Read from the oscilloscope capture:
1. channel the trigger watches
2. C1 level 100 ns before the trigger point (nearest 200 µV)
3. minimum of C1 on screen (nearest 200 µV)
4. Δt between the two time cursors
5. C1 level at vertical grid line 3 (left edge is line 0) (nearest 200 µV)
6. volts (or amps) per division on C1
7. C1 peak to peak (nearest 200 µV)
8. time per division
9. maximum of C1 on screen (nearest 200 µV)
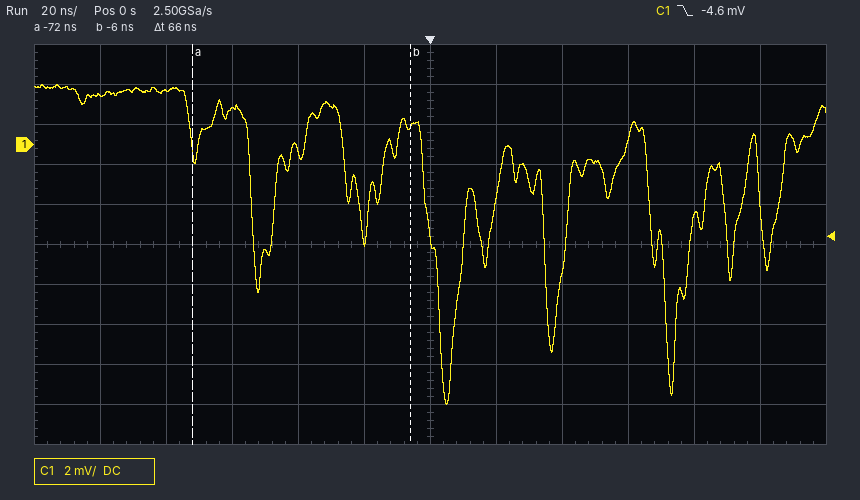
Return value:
C1
2.4 mV
-13.0 mV
66 ns
1.8 mV
2 mV
16.0 mV
20 ns
3.0 mV
